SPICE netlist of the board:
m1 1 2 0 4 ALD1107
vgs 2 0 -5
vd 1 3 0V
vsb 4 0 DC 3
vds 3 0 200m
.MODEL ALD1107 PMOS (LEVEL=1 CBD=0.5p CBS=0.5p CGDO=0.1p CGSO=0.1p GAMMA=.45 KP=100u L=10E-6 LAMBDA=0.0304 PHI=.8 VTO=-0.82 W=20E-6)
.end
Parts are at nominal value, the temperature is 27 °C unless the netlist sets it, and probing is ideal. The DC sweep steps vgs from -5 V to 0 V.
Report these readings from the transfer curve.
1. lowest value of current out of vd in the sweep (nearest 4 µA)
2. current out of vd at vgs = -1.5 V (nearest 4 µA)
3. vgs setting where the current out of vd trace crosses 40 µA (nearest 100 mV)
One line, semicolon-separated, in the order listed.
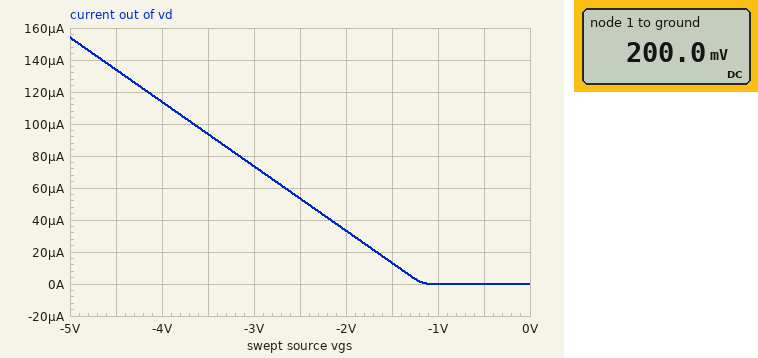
0 A; 12 µA; -2.2 V
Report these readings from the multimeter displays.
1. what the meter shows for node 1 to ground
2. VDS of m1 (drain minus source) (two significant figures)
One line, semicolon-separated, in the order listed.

200.0 mV; 200 mV
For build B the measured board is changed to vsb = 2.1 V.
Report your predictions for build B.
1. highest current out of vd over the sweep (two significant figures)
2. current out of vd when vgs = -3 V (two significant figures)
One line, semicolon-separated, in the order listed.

160 µA; 78 µA
